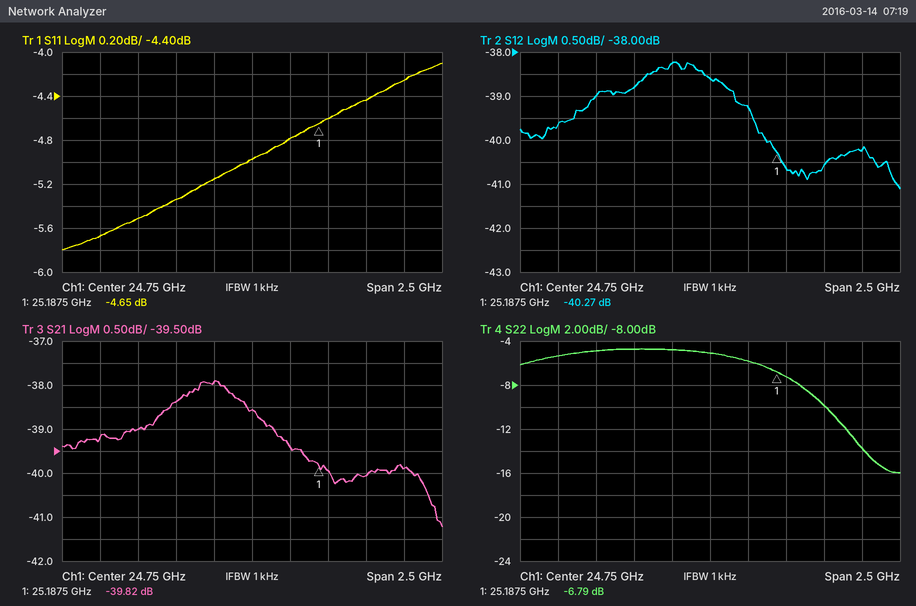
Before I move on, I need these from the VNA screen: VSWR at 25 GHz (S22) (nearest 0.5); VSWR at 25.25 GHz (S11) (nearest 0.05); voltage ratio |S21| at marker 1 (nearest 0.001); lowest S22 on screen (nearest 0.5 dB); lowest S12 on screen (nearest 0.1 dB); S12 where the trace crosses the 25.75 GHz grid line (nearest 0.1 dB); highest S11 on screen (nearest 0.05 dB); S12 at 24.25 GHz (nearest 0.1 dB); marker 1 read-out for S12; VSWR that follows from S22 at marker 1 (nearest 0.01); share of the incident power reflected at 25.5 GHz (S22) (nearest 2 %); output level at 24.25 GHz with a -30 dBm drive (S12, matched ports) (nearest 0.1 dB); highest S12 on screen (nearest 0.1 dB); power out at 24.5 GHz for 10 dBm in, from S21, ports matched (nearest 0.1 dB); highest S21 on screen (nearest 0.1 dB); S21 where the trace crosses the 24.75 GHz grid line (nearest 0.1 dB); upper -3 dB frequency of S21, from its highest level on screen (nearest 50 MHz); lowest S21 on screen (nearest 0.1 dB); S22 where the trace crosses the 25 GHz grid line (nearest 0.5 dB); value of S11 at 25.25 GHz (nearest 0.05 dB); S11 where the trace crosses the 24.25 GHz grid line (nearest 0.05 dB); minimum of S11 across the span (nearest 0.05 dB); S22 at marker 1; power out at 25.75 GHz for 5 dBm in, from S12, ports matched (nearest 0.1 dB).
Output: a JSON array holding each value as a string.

["3.0", "3.85", "0.010", "-16.0 dB", "-41.1 dB", "-40.2 dB", "-4.10 dB", "-38.8 dB", "-40.27 dB", "2.69", "10 %", "-68.8 dBm", "-38.2 dB", "-27.9 dBm", "-37.9 dB", "-38.6 dB", "25.95 GHz", "-41.2 dB", "-6.0 dB", "-4.60 dB", "-5.35 dB", "-5.80 dB", "-6.79 dB", "-35.2 dBm"]
